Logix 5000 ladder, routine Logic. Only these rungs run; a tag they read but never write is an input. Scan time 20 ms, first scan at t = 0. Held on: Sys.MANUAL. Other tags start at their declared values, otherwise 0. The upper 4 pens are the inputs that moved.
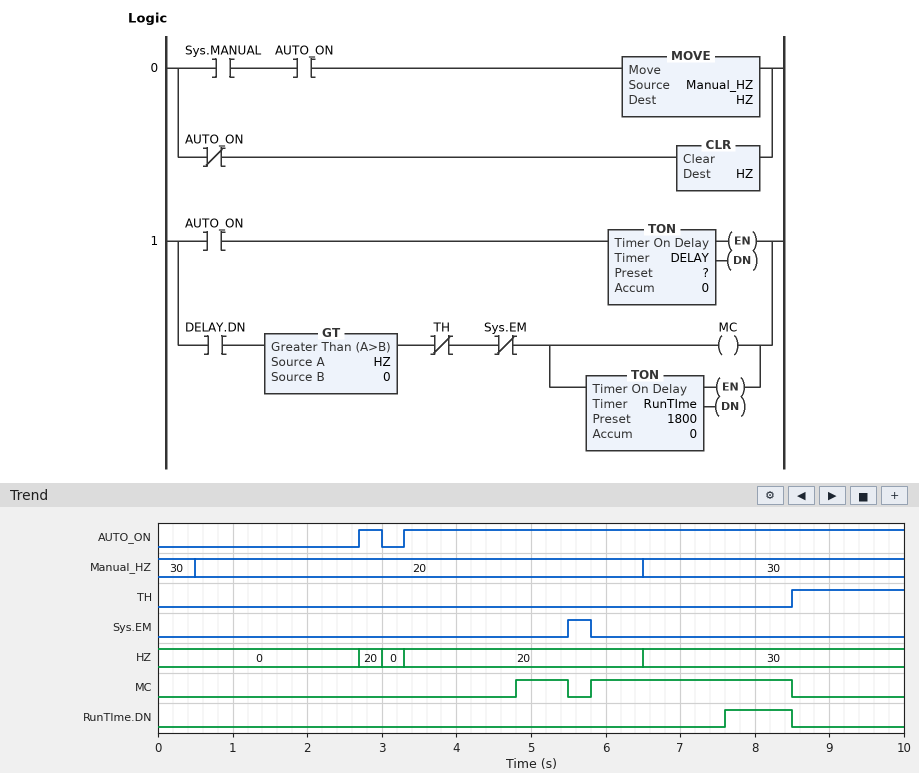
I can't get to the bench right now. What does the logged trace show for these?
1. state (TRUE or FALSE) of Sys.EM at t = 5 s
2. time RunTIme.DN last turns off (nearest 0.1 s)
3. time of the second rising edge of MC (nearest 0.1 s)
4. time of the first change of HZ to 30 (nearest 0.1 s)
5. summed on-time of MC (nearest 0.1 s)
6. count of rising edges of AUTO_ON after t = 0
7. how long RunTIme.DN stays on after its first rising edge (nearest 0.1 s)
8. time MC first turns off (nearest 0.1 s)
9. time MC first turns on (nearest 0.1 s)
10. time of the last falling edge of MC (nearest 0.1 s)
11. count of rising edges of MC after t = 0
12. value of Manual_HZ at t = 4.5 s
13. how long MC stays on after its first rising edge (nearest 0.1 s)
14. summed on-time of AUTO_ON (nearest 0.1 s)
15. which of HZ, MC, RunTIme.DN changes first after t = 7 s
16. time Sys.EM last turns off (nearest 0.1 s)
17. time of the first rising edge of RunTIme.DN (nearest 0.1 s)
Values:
FALSE
8.5 s
5.8 s
6.5 s
3.4 s
2
0.9 s
5.5 s
4.8 s
8.5 s
2
20
0.7 s
7.0 s
RunTIme.DN
5.8 s
7.6 s
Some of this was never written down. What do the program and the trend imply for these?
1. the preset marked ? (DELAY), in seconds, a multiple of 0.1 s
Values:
1.5 s
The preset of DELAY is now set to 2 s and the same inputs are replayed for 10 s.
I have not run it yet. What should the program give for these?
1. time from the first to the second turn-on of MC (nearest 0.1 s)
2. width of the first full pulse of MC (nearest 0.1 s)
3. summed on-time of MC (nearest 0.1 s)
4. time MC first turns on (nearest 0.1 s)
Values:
0.5 s
0.2 s
2.9 s
5.3 s
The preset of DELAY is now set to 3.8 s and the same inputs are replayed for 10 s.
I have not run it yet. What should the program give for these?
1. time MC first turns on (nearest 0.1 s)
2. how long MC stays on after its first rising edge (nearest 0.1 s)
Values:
7.1 s
1.4 s
